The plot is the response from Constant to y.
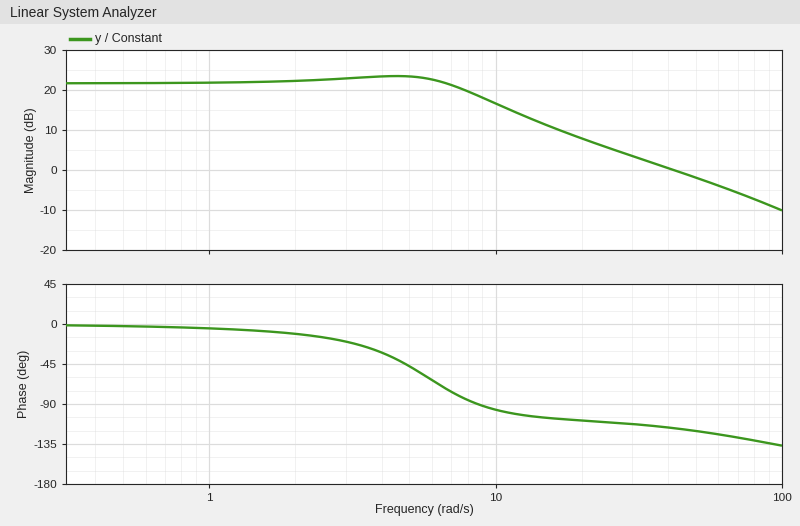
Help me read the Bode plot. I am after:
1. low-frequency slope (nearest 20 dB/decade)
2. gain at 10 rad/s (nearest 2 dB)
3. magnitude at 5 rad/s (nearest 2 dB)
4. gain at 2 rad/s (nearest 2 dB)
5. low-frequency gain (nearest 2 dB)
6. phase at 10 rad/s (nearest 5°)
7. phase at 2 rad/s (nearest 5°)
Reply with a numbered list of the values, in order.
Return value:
1. 0 dB/decade
2. 16 dB
3. 24 dB
4. 22 dB
5. 22 dB
6. -95°
7. -10°
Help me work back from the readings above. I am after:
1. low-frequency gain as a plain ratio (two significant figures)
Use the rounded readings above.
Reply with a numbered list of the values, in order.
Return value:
1. 13
